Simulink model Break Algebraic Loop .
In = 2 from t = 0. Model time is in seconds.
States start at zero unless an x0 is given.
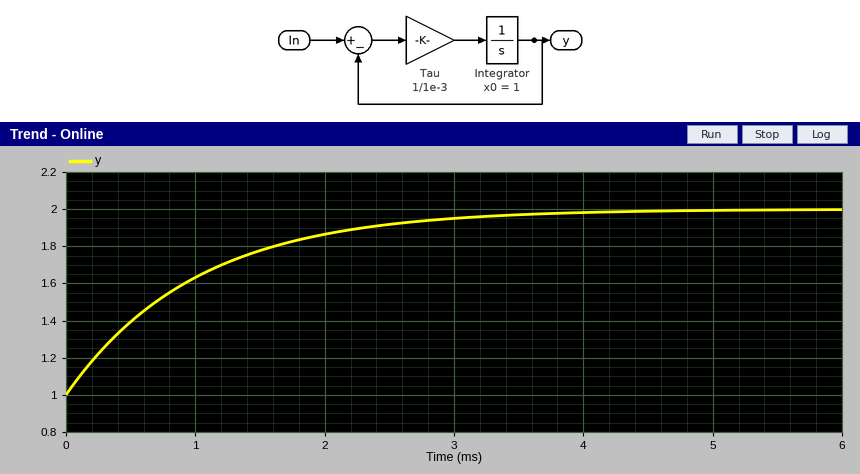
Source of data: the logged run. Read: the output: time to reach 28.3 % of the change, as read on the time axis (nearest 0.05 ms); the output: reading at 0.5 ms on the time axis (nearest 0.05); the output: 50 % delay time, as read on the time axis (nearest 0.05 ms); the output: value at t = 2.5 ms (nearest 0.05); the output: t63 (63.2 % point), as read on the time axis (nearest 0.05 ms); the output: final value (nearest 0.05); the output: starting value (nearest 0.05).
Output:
0.35 ms
1.40
0.70 ms
1.90
1.00 ms
2.00
1.00
